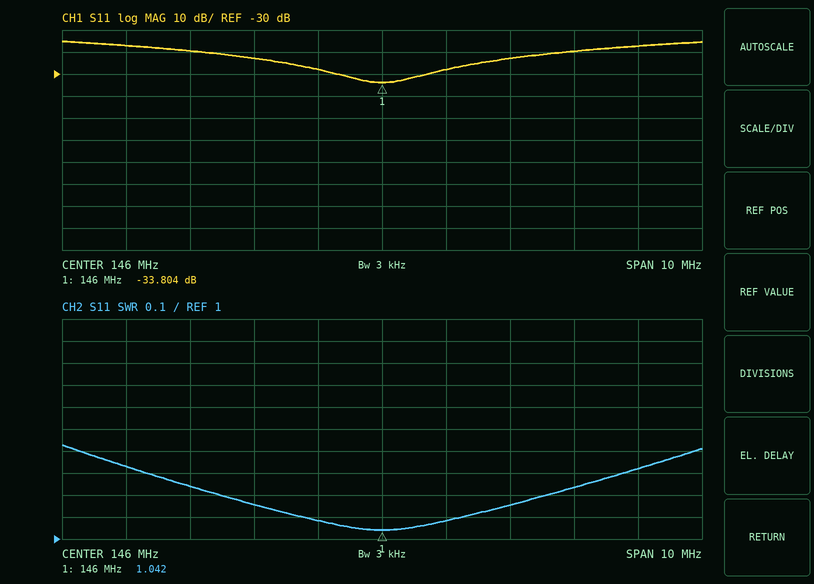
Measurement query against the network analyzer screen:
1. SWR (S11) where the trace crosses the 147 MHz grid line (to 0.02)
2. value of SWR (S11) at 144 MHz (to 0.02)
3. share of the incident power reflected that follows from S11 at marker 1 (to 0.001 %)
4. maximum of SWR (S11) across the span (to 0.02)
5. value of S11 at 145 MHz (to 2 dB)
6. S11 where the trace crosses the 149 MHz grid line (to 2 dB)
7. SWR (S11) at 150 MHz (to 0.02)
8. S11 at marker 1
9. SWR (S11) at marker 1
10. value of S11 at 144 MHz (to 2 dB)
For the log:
1.08
1.16
0.042 %
1.42
-28 dB
-20 dB
1.32
-33.804 dB
1.042
-22 dB
